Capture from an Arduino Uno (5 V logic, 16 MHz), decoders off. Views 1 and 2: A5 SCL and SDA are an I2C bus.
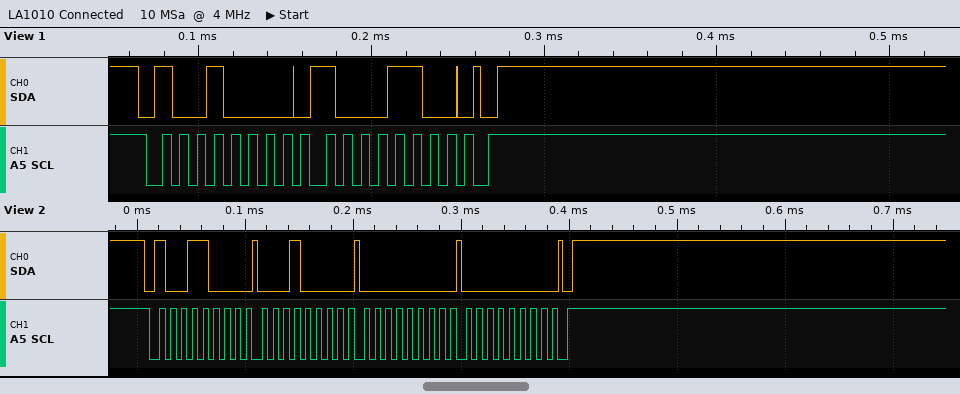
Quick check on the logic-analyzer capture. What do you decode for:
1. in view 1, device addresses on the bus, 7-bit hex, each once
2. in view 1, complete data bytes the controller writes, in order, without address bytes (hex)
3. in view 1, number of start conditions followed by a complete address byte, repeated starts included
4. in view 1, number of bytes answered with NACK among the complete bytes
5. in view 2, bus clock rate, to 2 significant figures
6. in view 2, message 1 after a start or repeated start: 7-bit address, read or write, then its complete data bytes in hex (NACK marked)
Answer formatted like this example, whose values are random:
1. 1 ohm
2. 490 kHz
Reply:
1. 0x48
2. 8C
3. 1
4. 0
5. 100 kHz
6. 0x4C write: 10 00 00
